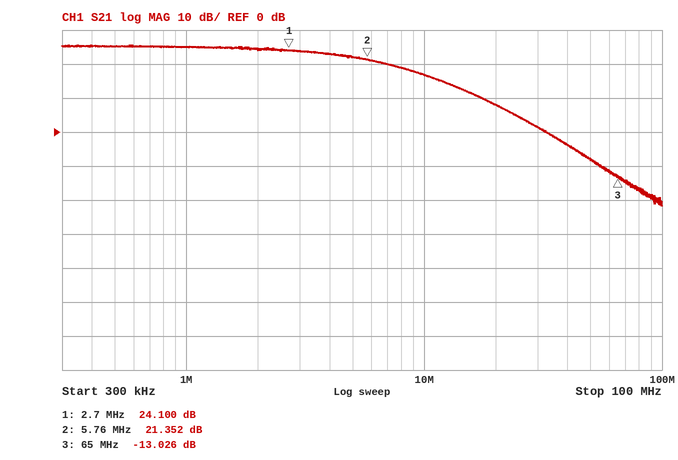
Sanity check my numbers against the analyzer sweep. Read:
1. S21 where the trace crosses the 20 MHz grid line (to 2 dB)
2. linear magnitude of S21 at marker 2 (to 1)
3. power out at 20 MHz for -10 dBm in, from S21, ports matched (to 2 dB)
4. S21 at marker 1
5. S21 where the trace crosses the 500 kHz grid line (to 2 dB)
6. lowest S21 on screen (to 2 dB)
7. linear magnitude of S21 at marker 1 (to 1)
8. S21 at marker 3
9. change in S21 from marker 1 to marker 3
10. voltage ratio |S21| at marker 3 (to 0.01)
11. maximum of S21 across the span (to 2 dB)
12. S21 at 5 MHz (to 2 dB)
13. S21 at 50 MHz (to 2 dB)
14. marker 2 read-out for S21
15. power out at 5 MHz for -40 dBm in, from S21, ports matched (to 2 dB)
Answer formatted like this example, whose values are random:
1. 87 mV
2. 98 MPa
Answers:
1. 8 dB
2. 12
3. -2 dBm
4. 24.100 dB
5. 26 dB
6. -22 dB
7. 16
8. -13.026 dB
9. -37.126 dB
10. 0.22
11. 26 dB
12. 22 dB
13. -8 dB
14. 21.352 dB
15. -18 dBm
